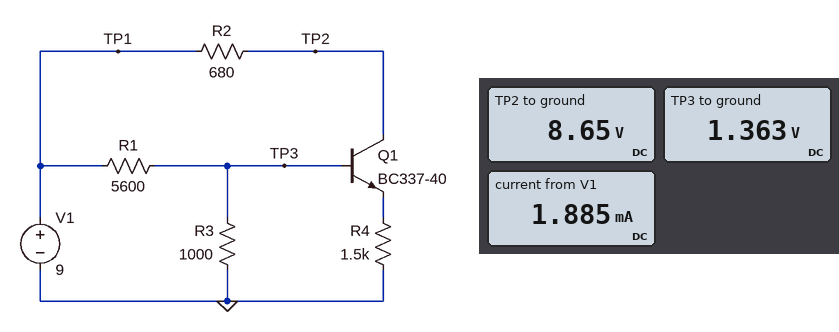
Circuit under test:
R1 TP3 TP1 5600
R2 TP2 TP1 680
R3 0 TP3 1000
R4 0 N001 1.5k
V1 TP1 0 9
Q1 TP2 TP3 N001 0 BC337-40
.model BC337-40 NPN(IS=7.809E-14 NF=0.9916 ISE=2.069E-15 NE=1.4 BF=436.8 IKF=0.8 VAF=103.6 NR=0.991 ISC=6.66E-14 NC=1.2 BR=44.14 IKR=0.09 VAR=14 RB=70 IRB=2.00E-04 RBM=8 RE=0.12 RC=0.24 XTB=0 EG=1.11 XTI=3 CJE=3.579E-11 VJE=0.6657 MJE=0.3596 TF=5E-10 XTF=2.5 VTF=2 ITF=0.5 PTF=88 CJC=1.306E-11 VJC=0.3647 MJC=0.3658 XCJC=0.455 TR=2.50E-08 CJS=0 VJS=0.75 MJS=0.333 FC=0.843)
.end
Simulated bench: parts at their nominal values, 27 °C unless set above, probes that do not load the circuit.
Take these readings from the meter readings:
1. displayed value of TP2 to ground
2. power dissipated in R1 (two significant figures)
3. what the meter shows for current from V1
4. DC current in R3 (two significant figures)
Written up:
8.65 V
10 mW
1.885 mA
1.4 mA
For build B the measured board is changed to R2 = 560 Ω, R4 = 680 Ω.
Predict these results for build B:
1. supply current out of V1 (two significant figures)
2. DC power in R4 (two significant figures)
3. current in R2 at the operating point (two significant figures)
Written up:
2.5 mA
850 µW
1.1 mA
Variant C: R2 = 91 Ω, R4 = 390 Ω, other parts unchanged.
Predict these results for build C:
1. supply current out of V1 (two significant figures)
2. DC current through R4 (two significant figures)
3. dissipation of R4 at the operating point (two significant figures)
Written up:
3.3 mA
1.9 mA
1.4 mW
